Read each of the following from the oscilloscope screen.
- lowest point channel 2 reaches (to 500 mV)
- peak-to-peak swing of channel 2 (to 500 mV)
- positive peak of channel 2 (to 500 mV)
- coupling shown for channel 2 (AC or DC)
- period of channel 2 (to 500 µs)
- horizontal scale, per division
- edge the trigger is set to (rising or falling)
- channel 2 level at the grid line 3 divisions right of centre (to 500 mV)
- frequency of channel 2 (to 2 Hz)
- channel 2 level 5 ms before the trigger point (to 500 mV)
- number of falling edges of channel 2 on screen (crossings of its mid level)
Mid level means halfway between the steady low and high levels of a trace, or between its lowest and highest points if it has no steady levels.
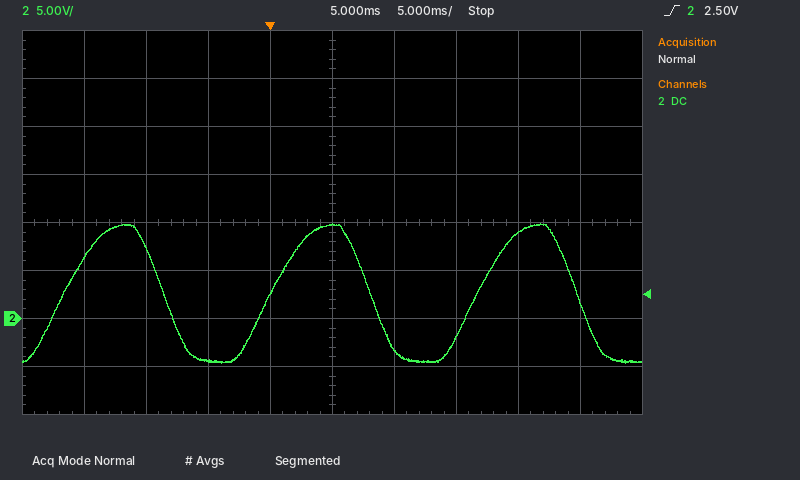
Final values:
-4.5 V
14.5 V
10.0 V
DC
16.5 ms
5 ms
rising
9.0 V
60 Hz
-4.5 V
3
